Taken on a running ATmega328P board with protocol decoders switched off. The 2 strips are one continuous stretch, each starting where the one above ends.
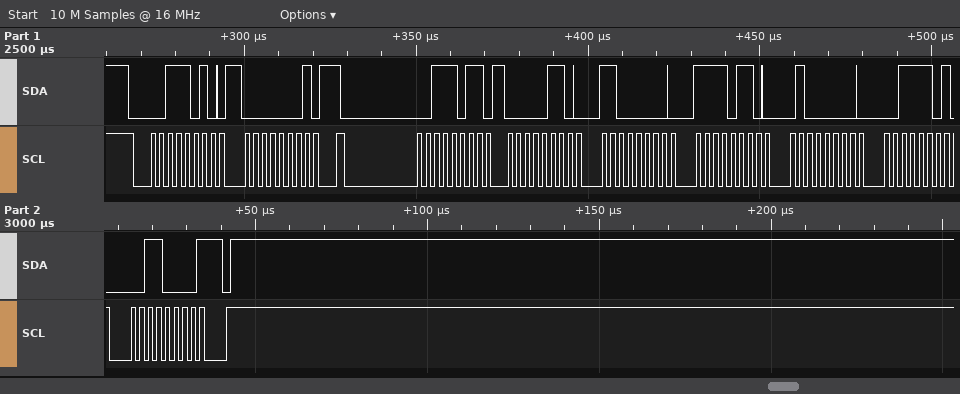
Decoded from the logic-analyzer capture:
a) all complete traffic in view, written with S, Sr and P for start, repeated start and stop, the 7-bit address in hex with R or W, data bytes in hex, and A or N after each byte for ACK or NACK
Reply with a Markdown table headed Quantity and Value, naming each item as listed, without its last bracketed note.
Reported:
| Quantity | Value |
|---|---|
| all complete traffic in view, written with S, Sr and P for start, repeated start and stop, the 7-bit address in hex with R or W, data bytes in hex, and A or N after each byte for ACK or NACK | S 1DW A 01 A Sr 1DR A 06 A C0 A F6 A 40 A 3D A 30 N P |
